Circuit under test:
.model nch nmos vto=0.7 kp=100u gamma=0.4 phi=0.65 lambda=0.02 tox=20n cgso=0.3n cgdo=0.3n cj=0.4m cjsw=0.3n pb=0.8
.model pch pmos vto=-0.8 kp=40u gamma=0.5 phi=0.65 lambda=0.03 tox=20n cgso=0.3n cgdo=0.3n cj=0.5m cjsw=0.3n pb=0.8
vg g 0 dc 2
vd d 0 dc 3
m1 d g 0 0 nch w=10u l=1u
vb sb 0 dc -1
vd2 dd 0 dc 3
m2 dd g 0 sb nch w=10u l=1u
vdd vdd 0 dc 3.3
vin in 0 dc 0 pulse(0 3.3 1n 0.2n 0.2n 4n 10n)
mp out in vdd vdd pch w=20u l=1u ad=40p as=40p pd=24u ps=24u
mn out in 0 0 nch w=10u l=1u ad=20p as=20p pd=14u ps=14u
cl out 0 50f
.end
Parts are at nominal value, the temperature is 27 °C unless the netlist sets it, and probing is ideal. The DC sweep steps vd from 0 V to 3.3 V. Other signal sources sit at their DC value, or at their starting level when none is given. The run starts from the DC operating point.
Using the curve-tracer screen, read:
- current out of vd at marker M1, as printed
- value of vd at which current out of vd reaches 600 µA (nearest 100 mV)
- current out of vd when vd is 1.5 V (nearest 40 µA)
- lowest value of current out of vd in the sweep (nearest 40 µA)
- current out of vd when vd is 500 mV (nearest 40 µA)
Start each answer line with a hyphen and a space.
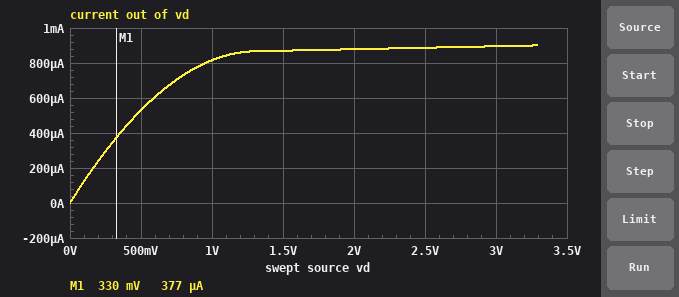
- 377 µA
- 600 mV
- 880 µA
- 0 A
- 520 µA
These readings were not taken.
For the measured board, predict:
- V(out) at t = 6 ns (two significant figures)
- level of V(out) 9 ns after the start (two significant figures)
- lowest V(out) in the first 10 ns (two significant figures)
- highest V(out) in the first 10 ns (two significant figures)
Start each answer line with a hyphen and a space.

- 3.3 V
- 3.3 V
- -120 mV
- 3.5 V
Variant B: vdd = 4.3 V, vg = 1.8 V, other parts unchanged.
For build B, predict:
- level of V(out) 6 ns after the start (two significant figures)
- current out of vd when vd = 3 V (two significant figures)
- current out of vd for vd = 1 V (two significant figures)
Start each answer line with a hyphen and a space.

- 4.3 V
- 640 µA
- 610 µA
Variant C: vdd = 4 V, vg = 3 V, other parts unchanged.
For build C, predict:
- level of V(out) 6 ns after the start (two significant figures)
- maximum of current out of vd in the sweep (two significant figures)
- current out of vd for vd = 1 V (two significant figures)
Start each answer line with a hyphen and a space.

- 4.0 V
- 2.8 mA
- 1.8 mA
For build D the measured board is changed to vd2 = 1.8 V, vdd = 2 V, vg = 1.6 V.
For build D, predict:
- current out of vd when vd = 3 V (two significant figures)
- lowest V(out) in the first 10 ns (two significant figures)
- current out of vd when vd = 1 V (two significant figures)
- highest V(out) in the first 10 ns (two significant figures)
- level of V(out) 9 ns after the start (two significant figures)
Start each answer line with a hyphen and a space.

- 430 µA
- -280 mV
- 410 µA
- 2.3 V
- 2.0 V
